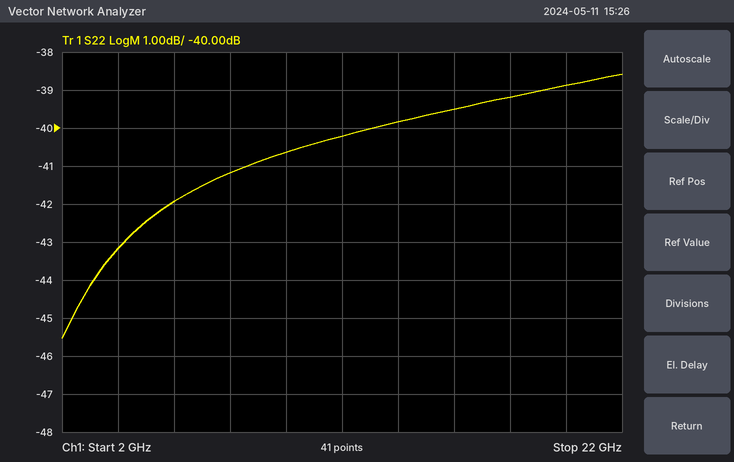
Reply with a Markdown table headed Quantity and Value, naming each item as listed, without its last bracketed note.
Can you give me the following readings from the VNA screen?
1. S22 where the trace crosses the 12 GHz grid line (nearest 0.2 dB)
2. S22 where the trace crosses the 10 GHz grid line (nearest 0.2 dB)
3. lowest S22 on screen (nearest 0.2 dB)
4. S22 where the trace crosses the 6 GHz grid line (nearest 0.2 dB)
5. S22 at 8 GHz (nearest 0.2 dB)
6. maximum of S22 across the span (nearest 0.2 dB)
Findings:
| Quantity | Value |
|---|---|
| S22 where the trace crosses the 12 GHz grid line | -40.2 dB |
| S22 where the trace crosses the 10 GHz grid line | -40.6 dB |
| lowest S22 on screen | -45.6 dB |
| S22 where the trace crosses the 6 GHz grid line | -42.0 dB |
| S22 at 8 GHz | -41.2 dB |
| maximum of S22 across the span | -38.6 dB |
